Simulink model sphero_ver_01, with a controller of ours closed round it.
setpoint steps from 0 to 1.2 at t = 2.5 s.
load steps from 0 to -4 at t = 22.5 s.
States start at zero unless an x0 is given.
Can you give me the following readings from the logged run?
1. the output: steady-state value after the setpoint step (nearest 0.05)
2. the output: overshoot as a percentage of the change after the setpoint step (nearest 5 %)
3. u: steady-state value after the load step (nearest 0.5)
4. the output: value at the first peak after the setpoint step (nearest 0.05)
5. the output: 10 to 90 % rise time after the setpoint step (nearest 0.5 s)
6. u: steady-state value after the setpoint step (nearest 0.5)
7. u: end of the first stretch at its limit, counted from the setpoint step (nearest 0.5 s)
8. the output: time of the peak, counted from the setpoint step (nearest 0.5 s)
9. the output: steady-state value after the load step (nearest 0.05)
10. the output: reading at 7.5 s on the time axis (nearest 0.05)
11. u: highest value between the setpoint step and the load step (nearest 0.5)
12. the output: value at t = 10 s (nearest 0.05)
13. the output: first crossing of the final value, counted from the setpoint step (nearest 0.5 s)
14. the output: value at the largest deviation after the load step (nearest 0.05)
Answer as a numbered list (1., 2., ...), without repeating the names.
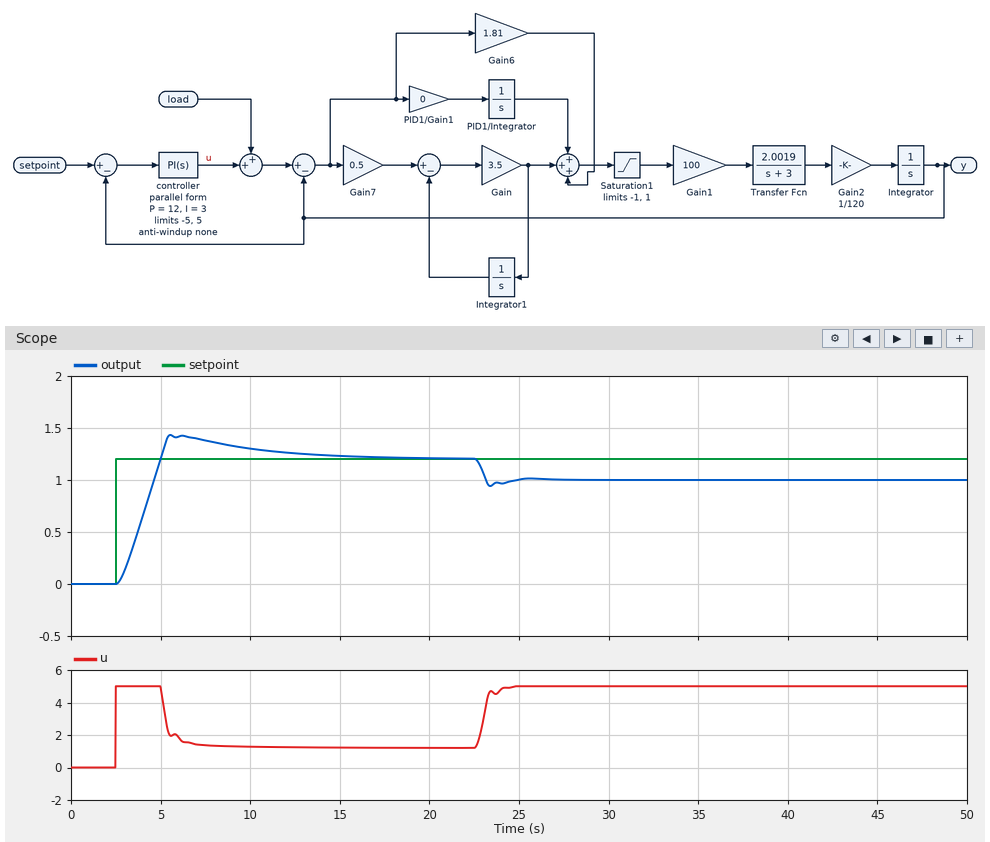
1. 1.20
2. 20 %
3. 5.0
4. 1.45
5. 2.0 s
6. 1.0
7. 2.5 s
8. 3.0 s
9. 1.00
10. 1.40
11. 5.0
12. 1.30
13. 2.5 s
14. 0.95
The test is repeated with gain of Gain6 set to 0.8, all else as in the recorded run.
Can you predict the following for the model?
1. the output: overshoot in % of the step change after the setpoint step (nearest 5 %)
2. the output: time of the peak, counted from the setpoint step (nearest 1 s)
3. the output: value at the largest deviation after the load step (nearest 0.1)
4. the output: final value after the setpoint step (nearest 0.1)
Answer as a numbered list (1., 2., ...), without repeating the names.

1. 15 %
2. 4 s
3. 1.0
4. 1.2
